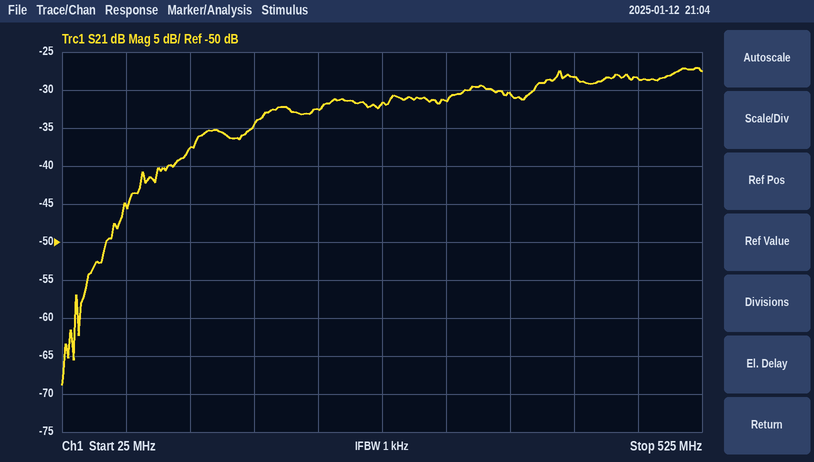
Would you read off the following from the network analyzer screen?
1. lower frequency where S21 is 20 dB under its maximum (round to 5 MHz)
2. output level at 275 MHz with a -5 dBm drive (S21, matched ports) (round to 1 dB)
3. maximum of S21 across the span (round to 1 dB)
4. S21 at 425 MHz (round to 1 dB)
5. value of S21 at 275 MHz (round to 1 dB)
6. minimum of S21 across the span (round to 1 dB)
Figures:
70 MHz
-37 dBm
-27 dB
-28 dB
-32 dB
-69 dB
